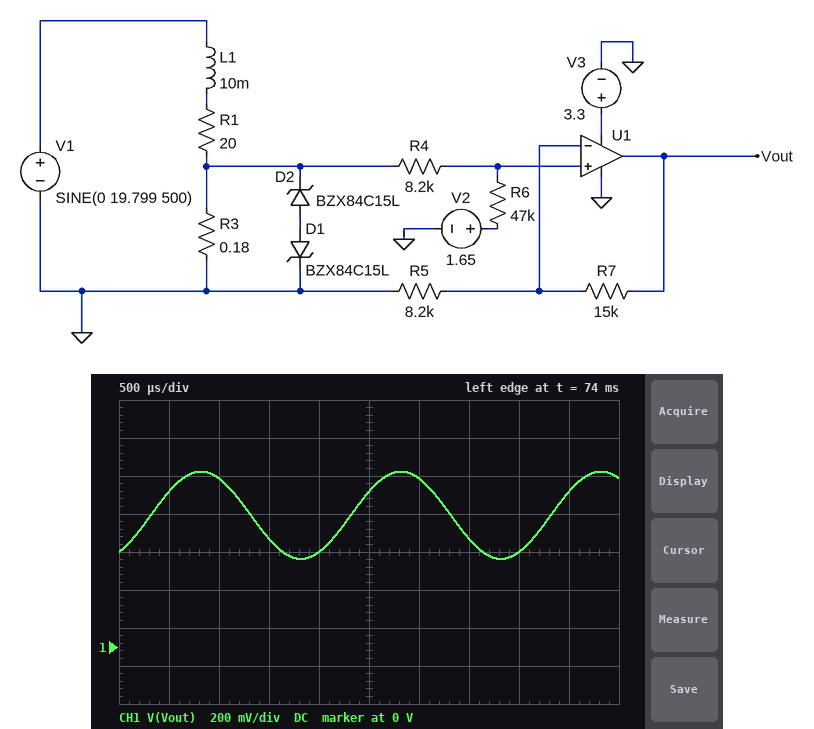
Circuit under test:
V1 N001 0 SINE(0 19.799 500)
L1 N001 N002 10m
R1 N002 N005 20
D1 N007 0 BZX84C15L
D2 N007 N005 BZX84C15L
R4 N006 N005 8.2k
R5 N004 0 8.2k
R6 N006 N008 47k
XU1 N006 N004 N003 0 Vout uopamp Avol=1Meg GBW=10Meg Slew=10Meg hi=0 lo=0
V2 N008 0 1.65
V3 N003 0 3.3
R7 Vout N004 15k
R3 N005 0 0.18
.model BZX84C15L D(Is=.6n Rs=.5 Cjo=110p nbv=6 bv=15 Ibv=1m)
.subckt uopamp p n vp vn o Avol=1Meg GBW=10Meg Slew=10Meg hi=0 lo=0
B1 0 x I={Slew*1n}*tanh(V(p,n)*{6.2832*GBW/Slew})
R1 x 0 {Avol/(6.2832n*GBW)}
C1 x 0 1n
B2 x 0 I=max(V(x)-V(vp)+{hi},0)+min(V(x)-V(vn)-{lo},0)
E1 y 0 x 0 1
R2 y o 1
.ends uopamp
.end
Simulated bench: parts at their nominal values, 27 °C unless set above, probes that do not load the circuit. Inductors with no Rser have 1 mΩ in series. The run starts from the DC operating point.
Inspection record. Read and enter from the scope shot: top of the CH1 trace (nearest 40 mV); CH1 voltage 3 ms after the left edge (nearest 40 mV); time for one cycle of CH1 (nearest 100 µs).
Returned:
920 mV
880 mV
2.0 ms
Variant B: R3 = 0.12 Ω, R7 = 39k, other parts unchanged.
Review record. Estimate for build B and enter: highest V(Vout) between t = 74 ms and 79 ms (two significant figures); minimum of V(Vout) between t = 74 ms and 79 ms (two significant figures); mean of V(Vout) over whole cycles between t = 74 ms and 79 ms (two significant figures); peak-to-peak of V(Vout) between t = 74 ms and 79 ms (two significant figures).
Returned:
1.7 V
1.1 V
1.4 V
620 mV
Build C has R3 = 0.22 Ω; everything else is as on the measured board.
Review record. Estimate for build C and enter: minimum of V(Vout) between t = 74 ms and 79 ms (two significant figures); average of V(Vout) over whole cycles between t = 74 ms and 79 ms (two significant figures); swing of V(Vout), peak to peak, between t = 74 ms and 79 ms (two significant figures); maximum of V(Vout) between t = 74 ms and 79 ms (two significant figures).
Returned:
410 mV
690 mV
560 mV
970 mV
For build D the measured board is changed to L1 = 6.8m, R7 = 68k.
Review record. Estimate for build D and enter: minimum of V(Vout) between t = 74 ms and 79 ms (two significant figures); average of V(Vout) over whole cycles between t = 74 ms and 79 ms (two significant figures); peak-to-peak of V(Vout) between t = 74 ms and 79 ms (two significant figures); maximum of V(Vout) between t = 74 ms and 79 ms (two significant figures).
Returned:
1.3 V
2.3 V
1.9 V
3.2 V
